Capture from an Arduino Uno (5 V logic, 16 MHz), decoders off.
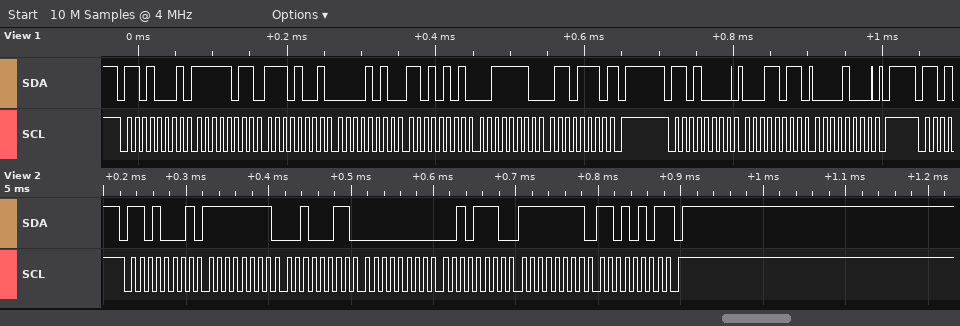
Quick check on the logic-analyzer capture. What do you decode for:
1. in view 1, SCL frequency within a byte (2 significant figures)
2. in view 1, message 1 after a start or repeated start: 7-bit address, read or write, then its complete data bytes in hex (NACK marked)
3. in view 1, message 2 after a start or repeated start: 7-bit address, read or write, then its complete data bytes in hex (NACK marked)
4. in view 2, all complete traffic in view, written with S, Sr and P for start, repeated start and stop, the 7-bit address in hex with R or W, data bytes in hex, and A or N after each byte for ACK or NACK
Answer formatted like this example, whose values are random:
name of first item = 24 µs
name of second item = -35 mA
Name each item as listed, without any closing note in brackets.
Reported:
in view 1, SCL frequency within a byte = 100 kHz
in view 1, message 1 after a start or repeated start: 7-bit address, read or write, then its complete data bytes in hex = 0x68 read: FB E9 0A D5 3E 6E NACK
in view 1, message 2 after a start or repeated start: 7-bit address, read or write, then its complete data bytes in hex = 0x68 write: 1B 08
in view 2, all complete traffic in view, written with S, Sr and P for start, repeated start and stop, the 7-bit address in hex with R or W, data bytes in hex, and A or N after each byte for ACK or NACK = S 68R A FF A 23 A 00 A 2E A FF A D5 N P
